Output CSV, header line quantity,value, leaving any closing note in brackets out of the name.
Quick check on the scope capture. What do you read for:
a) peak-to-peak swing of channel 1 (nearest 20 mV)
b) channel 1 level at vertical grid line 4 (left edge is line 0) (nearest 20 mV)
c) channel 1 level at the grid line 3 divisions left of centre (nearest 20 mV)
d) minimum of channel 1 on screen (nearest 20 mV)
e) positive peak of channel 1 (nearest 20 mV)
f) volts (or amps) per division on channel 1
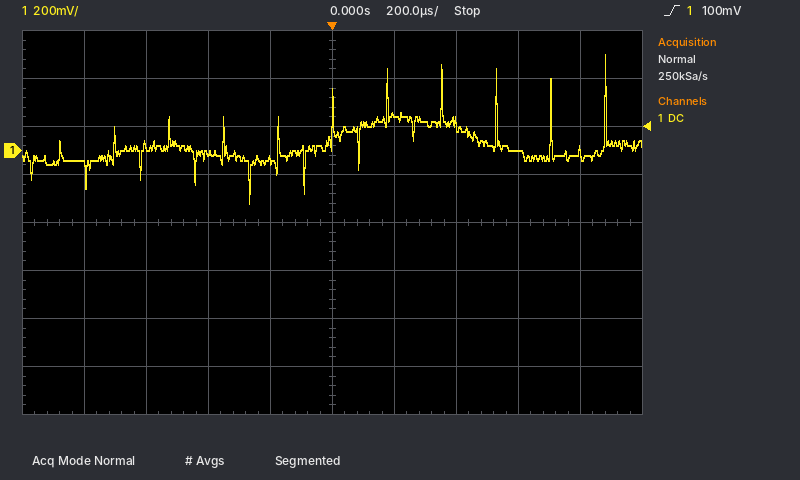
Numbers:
quantity,value
peak-to-peak swing of channel 1,620 mV
channel 1 level at vertical grid line 4 (left edge is line 0),-40 mV
channel 1 level at the grid line 3 divisions left of centre,20 mV
minimum of channel 1 on screen,-220 mV
positive peak of channel 1,400 mV
volts (or amps) per division on channel 1,200 mV
